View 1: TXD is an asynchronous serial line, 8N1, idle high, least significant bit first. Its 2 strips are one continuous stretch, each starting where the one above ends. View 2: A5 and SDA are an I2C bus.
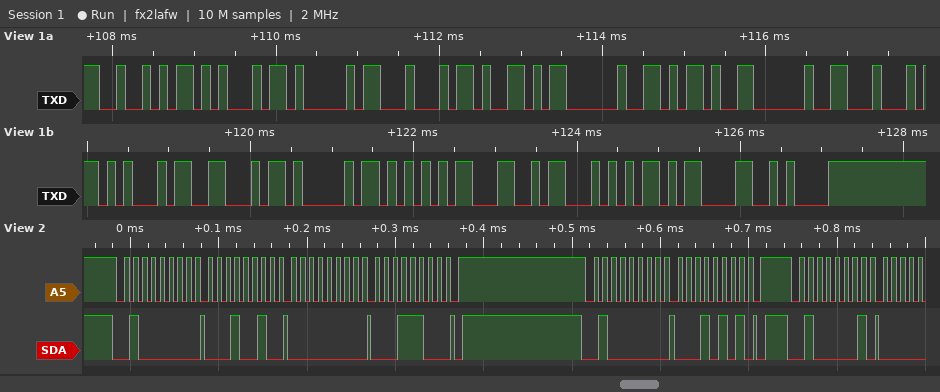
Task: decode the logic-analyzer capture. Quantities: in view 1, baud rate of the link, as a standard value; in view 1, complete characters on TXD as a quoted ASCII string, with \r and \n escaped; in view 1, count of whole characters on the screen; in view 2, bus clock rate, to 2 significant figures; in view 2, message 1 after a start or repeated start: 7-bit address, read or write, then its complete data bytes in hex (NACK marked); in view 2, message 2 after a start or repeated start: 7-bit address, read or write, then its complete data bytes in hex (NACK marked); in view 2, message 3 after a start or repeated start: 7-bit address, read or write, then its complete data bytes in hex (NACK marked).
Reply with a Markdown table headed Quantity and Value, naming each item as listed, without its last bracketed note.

| Quantity | Value |
|---|---|
| in view 1, baud rate of the link, as a standard value | 9600 baud |
| in view 1, complete characters on TXD as a quoted ASCII string, with \r and \n escaped | "READY - DEFAULT\r\n" |
| in view 1, count of whole characters on the screen | 17 |
| in view 2, bus clock rate, to 2 significant figures | 100 kHz |
| in view 2, message 1 after a start or repeated start: 7-bit address, read or write, then its complete data bytes in hex | 0x20 write: 12 00 1C |
| in view 2, message 2 after a start or repeated start: 7-bit address, read or write, then its complete data bytes in hex | 0x20 write: 15 |
| in view 2, message 3 after a start or repeated start: 7-bit address, read or write, then its complete data bytes in hex | 0x20 read |
